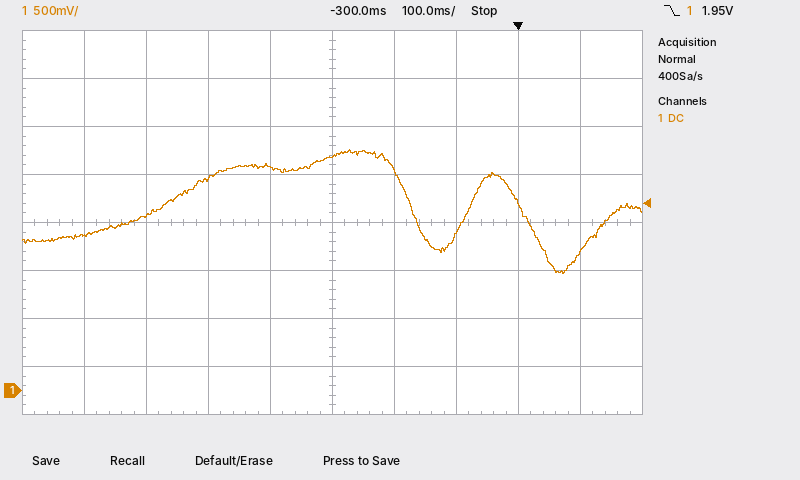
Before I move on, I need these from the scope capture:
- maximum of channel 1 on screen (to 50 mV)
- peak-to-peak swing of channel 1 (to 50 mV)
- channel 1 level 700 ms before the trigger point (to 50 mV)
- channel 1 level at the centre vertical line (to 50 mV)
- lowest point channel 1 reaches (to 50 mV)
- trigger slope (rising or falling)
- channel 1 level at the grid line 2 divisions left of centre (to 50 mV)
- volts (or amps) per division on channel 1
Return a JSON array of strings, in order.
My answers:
["2.50 V", "1.30 V", "1.60 V", "2.45 V", "1.20 V", "falling", "2.20 V", "500 mV"]
